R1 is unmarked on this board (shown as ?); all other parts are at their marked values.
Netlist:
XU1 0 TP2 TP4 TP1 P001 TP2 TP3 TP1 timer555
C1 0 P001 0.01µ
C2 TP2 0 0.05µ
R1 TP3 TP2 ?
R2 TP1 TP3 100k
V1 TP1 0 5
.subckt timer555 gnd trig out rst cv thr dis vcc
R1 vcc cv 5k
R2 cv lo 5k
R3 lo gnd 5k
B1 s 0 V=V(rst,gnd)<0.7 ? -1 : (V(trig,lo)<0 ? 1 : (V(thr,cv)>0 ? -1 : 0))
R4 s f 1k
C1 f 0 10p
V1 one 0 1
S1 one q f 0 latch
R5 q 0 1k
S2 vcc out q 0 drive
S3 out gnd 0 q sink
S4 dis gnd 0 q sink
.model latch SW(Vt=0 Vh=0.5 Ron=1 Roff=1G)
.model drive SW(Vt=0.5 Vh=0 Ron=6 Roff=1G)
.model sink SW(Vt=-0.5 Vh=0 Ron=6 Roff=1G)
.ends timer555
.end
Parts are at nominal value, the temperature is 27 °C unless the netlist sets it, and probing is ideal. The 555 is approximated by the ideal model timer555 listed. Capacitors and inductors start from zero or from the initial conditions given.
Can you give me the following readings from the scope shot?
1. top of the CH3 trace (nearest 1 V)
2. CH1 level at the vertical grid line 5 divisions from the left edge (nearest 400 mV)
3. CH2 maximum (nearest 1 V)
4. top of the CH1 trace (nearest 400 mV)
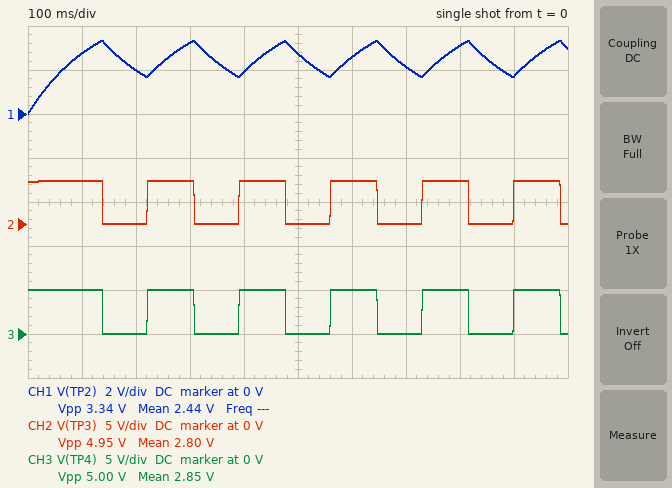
5 V
2.8 V
5 V
3.2 V
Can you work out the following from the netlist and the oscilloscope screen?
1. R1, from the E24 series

2.4 MΩ
